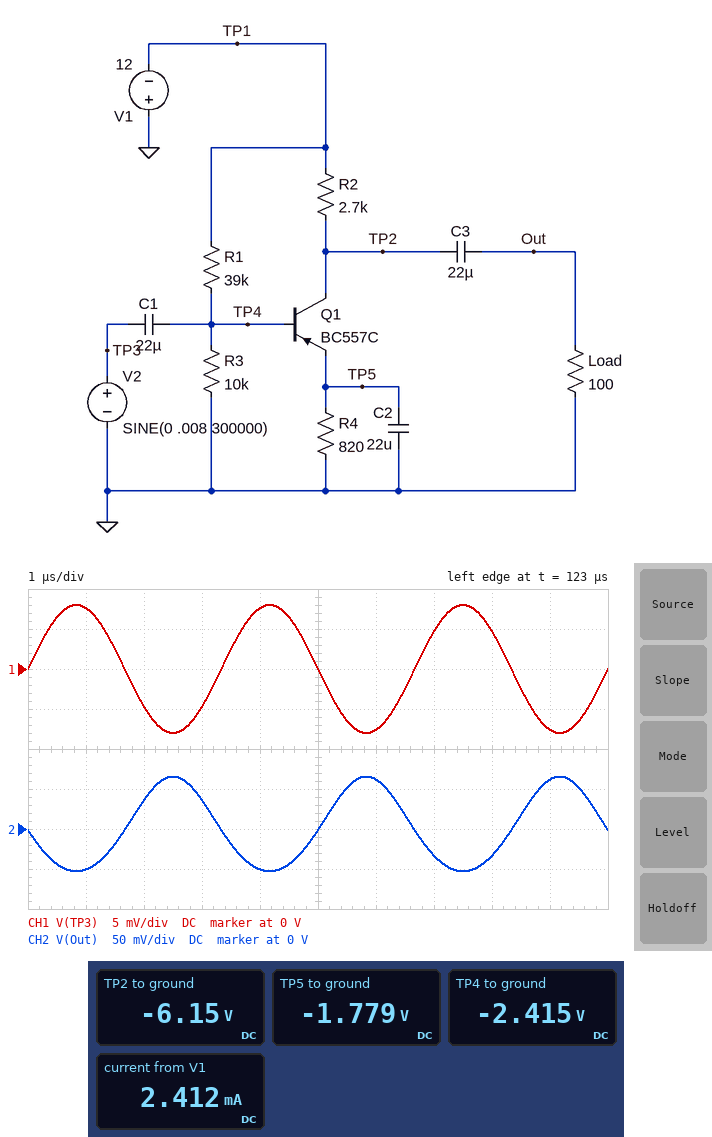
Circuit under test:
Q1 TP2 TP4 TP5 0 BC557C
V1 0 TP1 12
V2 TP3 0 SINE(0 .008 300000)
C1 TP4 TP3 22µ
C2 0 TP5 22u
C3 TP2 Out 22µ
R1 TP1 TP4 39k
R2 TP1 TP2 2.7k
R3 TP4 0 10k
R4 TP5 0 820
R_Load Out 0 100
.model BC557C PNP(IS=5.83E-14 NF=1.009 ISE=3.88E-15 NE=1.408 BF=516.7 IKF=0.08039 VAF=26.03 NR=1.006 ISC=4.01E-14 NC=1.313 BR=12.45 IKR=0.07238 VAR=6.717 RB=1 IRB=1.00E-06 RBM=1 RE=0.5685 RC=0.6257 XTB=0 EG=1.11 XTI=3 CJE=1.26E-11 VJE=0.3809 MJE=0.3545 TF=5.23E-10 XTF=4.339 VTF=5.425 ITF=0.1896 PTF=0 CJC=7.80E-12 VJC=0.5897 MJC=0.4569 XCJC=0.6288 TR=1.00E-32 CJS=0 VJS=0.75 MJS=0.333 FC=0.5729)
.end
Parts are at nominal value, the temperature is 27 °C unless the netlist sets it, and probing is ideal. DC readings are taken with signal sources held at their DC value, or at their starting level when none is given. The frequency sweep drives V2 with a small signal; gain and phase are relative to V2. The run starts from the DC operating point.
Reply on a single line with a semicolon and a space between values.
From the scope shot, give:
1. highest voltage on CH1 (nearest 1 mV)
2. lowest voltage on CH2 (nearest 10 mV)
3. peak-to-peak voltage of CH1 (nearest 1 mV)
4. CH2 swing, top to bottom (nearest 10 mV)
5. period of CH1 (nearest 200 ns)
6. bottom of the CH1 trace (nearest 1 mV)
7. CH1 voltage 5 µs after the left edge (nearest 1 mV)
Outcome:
8 mV; -50 mV; 16 mV; 120 mV; 3.4 µs; -8 mV; 0 V
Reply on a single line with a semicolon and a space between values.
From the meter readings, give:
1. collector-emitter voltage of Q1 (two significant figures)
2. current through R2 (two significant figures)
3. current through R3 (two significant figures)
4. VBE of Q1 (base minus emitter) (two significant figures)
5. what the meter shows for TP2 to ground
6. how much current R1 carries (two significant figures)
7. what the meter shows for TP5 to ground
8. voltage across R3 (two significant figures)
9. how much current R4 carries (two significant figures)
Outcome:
-4.4 V; 2.2 mA; 240 µA; -640 mV; -6.15 V; 250 µA; -1.779 V; 2.4 V; 2.2 mA
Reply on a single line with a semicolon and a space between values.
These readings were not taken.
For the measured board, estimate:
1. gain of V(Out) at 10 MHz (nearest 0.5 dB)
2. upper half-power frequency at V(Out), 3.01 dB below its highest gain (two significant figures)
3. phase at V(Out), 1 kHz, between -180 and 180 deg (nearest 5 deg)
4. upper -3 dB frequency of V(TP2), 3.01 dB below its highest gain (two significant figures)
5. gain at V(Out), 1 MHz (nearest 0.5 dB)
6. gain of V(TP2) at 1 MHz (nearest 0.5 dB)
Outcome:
17.5 dB; 470 MHz; -150 deg; 470 MHz; 17.5 dB; 17.5 dB
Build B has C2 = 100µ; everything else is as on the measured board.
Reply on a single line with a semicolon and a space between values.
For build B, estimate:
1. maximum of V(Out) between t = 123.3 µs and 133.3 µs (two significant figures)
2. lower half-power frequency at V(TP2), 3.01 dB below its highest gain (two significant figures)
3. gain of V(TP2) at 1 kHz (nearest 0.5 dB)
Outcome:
67 mV; 73 Hz; 17.5 dB
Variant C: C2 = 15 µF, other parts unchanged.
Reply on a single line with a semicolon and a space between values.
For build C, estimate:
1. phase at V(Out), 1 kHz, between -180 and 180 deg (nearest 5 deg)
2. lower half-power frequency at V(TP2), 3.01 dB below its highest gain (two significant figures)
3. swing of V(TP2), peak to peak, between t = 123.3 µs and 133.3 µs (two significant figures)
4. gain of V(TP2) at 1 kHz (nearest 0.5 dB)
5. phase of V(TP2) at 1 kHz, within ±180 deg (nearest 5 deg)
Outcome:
-140 deg; 820 Hz; 120 mV; 15.0 dB; -145 deg
